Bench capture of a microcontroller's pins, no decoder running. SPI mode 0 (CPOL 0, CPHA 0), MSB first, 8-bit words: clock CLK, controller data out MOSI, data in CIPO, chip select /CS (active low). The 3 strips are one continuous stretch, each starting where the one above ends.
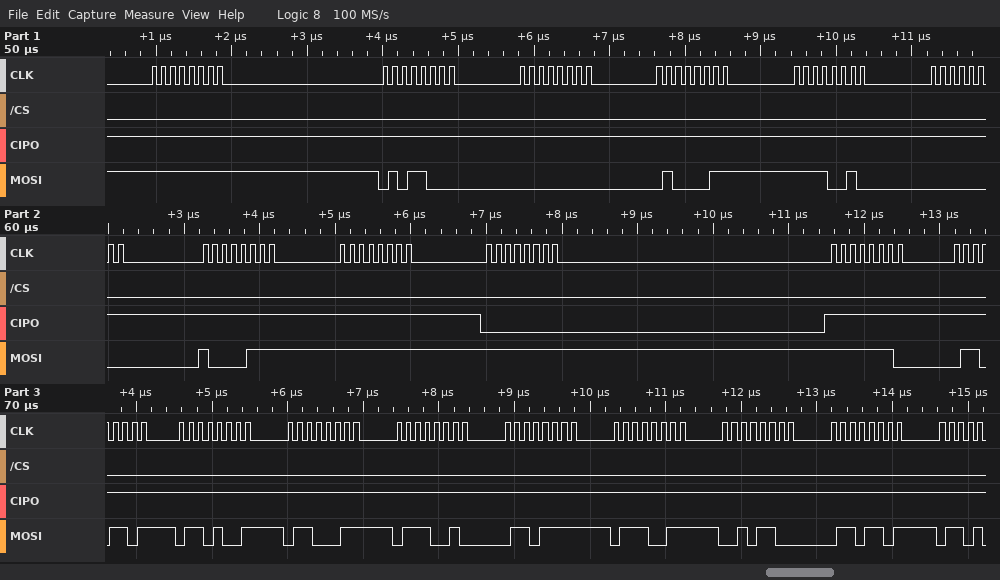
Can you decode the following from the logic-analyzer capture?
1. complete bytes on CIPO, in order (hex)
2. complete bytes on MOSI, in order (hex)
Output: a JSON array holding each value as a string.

["FF FF FF FF FF FF FF FF 00 FF FF FF FF FF FF FF FF FF", "FF 58 00 43 F2 00 87 FF FF FE 6D 69 63 72 6F 73 2C 6D"]
